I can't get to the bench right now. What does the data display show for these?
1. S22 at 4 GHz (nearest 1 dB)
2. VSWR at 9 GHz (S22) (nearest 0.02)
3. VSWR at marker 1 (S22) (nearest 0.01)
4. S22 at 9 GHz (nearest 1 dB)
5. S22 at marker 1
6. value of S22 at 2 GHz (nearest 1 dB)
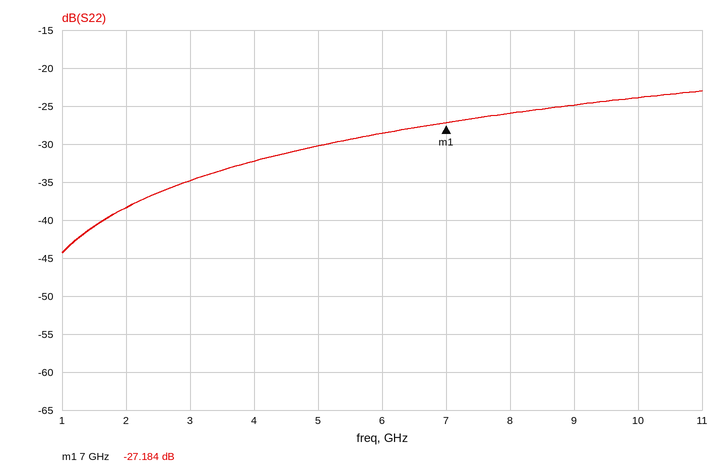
-32 dB
1.12
1.09
-25 dB
-27.184 dB
-38 dB
